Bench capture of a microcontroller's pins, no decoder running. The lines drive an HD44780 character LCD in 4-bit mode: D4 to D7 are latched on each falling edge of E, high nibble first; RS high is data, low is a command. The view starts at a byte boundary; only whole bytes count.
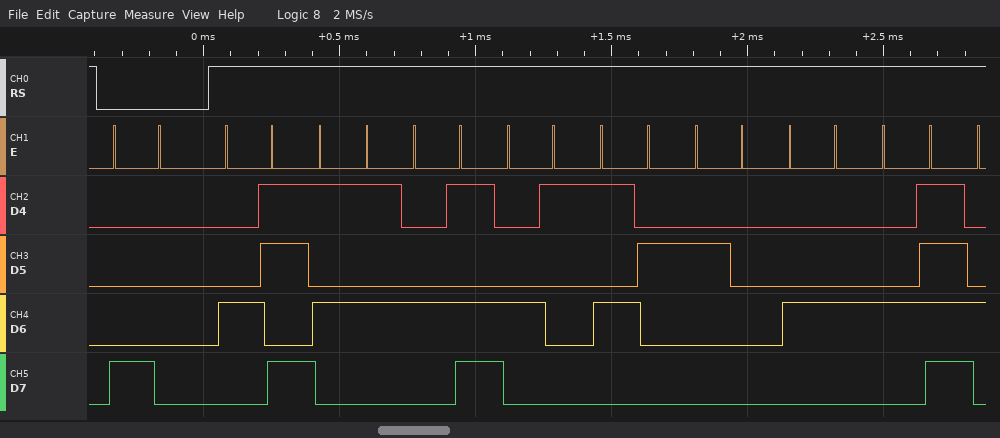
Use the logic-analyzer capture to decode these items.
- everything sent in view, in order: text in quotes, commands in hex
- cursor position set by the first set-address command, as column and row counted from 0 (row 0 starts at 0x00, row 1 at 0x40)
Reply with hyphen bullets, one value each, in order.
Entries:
- 0x80 "KUMAR DO"
- column 0, row 0
